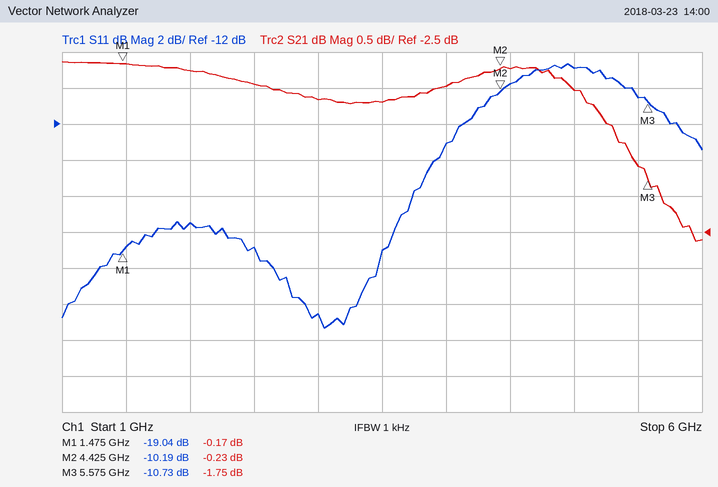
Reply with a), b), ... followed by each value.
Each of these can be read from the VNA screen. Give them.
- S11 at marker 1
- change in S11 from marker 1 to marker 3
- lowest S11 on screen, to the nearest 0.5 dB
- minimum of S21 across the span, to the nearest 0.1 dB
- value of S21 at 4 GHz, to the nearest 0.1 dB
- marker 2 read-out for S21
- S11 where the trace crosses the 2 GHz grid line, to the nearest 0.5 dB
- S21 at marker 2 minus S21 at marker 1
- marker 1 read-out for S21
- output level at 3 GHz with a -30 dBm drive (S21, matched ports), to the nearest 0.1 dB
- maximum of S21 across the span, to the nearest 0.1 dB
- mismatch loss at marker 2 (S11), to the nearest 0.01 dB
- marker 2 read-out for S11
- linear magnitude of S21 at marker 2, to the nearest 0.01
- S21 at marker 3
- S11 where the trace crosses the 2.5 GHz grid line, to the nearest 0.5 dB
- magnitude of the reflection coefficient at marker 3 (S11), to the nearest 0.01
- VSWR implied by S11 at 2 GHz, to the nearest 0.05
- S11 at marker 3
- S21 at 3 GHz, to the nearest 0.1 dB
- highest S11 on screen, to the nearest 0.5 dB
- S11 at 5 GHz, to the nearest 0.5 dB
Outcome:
a) -19.04 dB
b) 8.31 dB
c) -23.5 dB
d) -2.6 dB
e) -0.5 dB
f) -0.23 dB
g) -17.5 dB
h) -0.06 dB
i) -0.17 dB
j) -30.7 dBm
k) -0.1 dB
l) 0.44 dB
m) -10.19 dB
n) 0.97
o) -1.75 dB
p) -19.0 dB
q) 0.29
r) 1.30
s) -10.73 dB
t) -0.7 dB
u) -8.5 dB
v) -9.0 dB
